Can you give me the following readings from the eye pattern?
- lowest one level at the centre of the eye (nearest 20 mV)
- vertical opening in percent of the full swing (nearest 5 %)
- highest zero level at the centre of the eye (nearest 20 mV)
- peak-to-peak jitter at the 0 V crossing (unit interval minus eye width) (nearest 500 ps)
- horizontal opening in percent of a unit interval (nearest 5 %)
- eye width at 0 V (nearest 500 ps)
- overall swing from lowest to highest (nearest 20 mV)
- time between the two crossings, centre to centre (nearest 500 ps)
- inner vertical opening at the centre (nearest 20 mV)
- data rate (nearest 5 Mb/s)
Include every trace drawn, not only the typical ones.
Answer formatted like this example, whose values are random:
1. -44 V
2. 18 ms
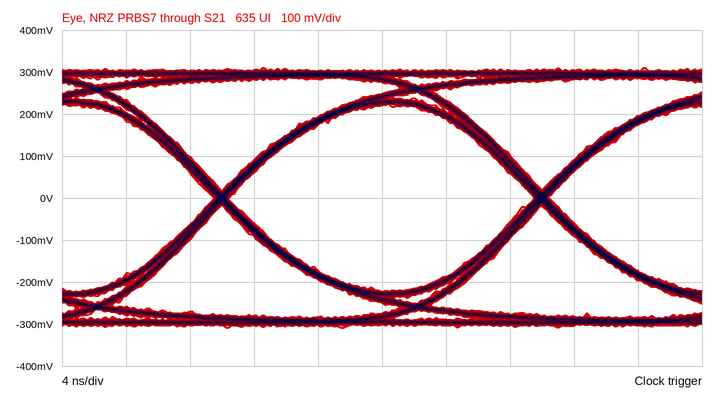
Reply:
1. 220 mV
2. 70 %
3. -220 mV
4. 1.0 ns
5. 95 %
6. 19.0 ns
7. 620 mV
8. 20.0 ns
9. 440 mV
10. 50 Mb/s
